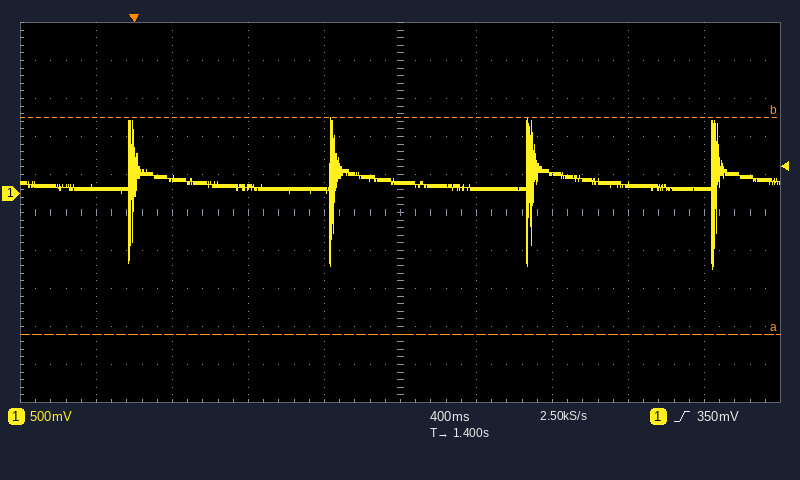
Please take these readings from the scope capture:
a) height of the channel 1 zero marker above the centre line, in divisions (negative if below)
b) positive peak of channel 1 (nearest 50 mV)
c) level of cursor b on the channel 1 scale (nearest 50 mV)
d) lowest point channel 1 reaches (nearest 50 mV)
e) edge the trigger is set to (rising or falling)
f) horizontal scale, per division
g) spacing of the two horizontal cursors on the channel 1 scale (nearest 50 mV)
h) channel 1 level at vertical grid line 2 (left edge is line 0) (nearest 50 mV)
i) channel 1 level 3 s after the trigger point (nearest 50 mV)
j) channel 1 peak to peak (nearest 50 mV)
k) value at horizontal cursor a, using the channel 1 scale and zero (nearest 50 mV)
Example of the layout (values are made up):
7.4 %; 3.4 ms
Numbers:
+0.5 div; 1.00 V; 1.00 V; -1.00 V; rising; 400 ms; 2.85 V; 200 mV; 50 mV; 2.00 V; -1.85 V
